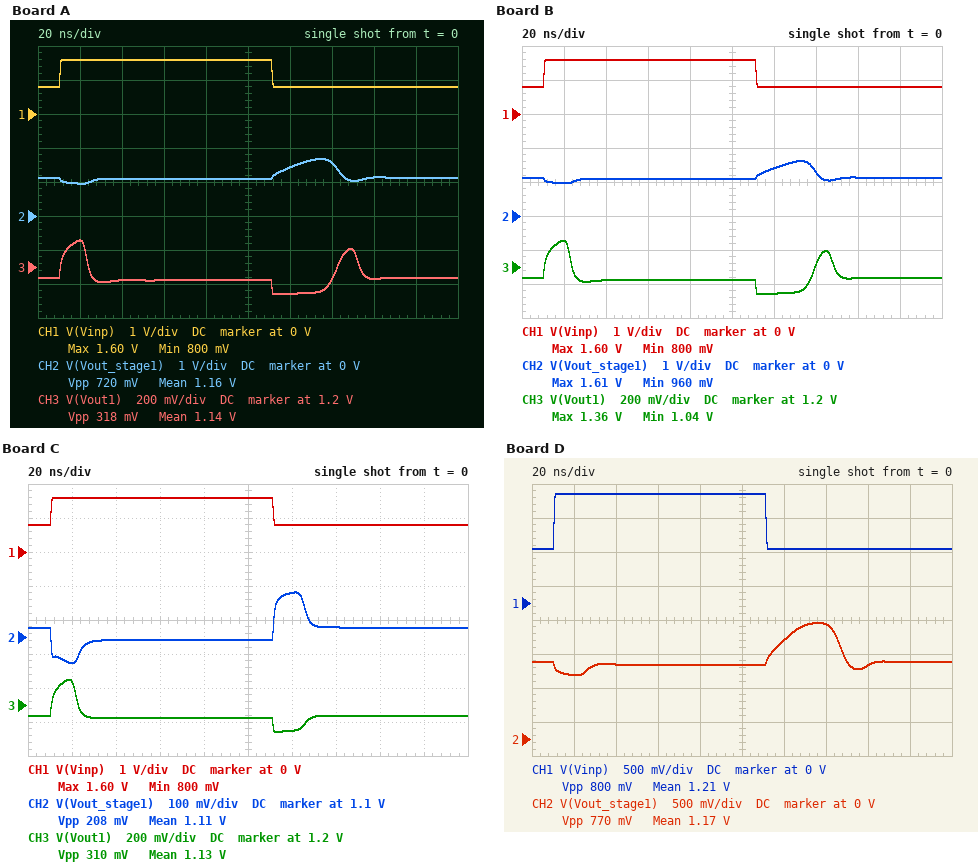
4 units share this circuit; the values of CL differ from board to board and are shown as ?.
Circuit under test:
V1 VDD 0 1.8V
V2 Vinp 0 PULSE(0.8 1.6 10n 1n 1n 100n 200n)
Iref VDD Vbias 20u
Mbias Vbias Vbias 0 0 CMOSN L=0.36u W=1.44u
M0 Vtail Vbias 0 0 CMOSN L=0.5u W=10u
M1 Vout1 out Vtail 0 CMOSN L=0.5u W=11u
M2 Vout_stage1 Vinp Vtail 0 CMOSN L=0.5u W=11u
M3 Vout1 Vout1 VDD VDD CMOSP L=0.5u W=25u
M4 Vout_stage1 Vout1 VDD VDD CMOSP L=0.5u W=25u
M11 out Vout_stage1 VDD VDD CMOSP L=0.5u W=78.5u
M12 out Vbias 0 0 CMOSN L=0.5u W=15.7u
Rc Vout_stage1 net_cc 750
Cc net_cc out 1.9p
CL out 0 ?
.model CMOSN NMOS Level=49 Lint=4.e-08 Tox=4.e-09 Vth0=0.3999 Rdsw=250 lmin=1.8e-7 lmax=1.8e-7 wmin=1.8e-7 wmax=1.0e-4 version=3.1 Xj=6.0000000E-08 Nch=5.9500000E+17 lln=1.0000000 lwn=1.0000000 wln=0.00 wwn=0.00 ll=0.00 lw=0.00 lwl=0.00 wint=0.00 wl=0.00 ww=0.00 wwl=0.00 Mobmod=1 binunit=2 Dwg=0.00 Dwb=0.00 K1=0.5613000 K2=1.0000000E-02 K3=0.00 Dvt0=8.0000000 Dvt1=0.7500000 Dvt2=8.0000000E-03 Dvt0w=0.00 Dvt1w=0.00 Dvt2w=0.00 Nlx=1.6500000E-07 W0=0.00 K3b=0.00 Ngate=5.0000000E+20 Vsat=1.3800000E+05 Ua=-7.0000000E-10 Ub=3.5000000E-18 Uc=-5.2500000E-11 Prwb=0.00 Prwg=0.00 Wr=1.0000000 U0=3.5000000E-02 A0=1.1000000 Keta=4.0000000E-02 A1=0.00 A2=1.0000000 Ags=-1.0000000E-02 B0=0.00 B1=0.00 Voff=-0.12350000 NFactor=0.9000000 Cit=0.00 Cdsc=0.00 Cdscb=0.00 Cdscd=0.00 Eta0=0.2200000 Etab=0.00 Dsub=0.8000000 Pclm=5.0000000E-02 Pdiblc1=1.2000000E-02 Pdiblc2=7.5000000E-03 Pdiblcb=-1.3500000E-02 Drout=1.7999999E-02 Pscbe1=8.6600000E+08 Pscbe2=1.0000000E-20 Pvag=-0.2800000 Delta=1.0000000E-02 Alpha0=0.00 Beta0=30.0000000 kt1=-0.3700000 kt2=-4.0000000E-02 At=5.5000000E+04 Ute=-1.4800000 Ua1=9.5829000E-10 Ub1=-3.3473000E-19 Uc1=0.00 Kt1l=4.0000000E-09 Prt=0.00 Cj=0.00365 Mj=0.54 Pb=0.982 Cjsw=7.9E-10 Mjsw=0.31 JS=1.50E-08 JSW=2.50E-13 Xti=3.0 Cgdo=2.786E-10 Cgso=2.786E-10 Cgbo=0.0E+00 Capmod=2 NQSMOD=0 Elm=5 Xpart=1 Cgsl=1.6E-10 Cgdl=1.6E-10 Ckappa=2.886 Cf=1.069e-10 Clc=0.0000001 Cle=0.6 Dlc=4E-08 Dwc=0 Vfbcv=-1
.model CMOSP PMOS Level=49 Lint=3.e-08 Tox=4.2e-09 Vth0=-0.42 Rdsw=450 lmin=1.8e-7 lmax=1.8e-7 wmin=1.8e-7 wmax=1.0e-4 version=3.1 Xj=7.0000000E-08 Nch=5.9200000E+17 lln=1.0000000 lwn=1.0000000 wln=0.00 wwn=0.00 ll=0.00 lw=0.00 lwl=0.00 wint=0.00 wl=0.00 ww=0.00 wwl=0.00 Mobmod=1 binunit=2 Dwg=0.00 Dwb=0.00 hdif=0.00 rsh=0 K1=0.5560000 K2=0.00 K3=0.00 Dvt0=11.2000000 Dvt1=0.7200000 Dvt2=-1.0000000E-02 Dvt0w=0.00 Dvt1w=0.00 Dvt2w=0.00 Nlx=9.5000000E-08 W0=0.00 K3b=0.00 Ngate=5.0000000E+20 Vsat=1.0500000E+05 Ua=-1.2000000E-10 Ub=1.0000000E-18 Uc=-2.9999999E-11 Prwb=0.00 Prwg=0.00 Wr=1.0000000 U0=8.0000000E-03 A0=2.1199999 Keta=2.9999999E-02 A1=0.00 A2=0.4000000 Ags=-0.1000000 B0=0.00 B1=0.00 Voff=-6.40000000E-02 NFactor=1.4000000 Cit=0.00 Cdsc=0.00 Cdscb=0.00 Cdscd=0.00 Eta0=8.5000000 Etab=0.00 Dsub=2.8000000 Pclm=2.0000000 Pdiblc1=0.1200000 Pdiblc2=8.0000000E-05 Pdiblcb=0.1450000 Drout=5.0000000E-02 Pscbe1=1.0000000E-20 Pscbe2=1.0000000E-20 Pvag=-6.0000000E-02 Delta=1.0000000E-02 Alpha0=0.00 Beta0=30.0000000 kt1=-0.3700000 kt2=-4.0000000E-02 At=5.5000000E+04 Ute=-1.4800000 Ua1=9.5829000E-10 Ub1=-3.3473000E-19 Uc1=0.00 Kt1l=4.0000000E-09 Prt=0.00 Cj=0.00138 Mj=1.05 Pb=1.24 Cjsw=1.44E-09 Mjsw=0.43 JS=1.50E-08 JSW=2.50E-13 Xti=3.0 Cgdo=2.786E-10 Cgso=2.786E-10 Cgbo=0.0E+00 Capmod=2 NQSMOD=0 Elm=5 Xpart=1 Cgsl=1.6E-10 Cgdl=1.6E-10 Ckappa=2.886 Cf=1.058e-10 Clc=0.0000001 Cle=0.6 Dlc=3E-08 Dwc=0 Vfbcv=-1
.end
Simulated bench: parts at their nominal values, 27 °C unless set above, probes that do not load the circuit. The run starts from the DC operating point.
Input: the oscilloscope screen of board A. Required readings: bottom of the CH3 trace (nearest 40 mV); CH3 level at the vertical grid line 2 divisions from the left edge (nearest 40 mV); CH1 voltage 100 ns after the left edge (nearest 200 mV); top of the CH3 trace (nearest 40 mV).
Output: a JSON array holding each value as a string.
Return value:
["1.04 V", "1.12 V", "1.6 V", "1.36 V"]
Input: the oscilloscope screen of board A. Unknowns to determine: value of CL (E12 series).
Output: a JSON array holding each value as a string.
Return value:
["3.9 pF"]
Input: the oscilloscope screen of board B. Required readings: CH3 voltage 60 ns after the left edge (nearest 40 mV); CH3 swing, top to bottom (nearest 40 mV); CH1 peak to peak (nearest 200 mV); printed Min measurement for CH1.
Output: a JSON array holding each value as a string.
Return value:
["1.12 V", "320 mV", "800 mV", "800 mV"]
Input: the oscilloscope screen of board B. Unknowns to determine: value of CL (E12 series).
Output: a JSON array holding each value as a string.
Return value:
["3.3 pF"]
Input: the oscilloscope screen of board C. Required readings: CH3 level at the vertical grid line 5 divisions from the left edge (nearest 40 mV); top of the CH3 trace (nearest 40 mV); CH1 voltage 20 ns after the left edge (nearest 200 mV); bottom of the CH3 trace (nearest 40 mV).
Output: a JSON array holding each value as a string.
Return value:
["1.12 V", "1.36 V", "1.6 V", "1.04 V"]
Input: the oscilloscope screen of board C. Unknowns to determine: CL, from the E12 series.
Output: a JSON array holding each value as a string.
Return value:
["680 fF"]
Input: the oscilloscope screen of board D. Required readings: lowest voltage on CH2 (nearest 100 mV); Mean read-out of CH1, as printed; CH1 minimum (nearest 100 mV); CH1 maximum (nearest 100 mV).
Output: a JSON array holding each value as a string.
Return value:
["900 mV", "1.21 V", "800 mV", "1.6 V"]
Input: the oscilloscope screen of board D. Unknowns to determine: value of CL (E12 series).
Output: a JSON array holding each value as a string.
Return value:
["4.7 pF"]
